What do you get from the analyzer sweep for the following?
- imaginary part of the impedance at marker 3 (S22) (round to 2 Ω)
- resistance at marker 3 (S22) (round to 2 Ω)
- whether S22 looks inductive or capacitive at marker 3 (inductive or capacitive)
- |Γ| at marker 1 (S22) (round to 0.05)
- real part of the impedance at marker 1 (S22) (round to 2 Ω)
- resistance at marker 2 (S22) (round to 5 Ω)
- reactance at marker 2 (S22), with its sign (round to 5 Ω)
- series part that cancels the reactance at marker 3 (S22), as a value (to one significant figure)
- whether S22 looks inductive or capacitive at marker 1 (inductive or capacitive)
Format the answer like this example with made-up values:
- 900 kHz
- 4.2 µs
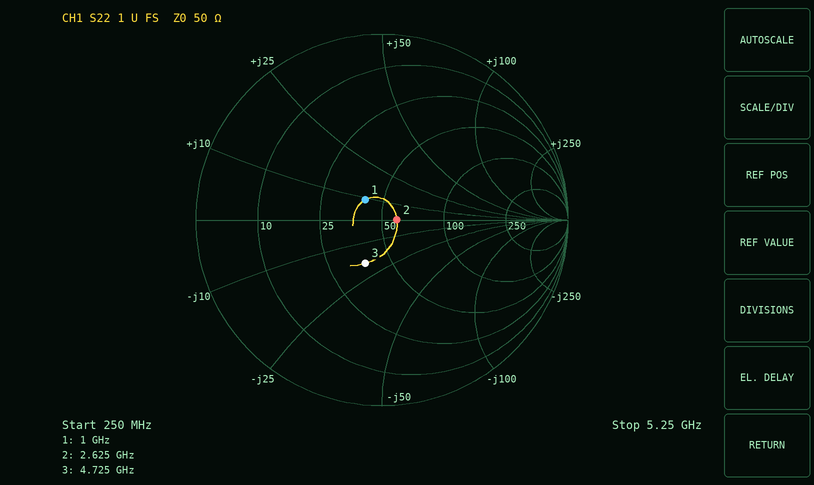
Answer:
- -18 Ω
- 38 Ω
- capacitive
- 0.15
- 40 Ω
- 60 Ω
- 0 Ω
- 600 pH
- inductive
